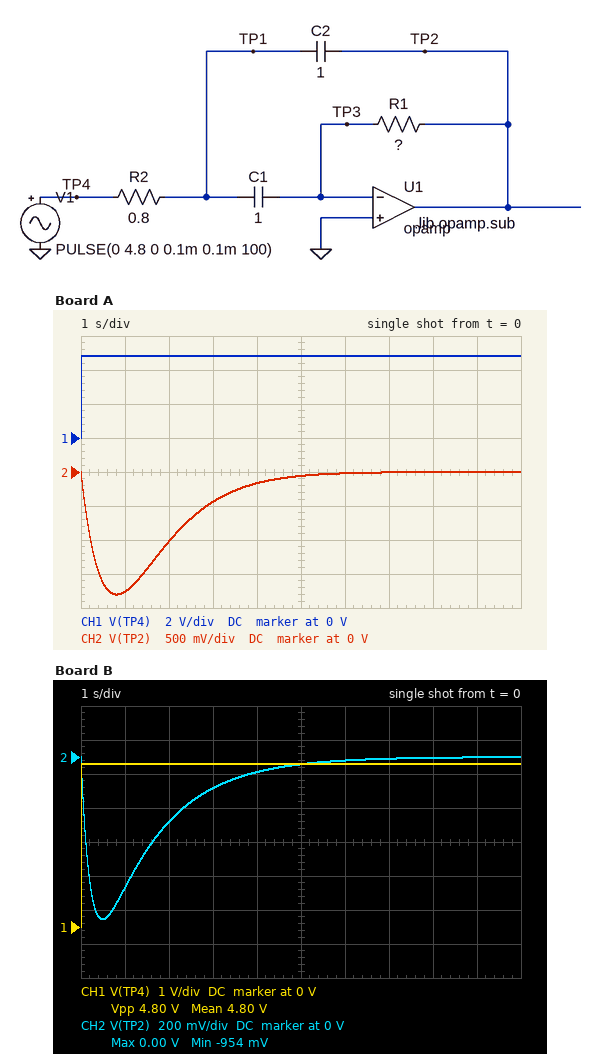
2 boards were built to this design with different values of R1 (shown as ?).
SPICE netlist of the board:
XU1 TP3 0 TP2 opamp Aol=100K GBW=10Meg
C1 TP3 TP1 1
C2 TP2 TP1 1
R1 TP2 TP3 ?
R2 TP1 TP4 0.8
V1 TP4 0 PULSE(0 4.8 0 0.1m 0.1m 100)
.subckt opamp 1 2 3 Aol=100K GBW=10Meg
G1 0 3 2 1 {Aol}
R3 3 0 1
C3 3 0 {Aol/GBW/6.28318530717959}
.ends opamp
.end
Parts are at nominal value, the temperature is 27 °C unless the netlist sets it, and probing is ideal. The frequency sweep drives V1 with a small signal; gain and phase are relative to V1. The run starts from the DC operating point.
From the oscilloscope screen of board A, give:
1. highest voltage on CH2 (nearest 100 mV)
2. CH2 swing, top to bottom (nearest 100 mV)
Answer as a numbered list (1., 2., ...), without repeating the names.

1. 0 V
2. 1.8 V
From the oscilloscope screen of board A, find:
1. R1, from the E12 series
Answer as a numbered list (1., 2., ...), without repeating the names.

1. 0.82 Ω
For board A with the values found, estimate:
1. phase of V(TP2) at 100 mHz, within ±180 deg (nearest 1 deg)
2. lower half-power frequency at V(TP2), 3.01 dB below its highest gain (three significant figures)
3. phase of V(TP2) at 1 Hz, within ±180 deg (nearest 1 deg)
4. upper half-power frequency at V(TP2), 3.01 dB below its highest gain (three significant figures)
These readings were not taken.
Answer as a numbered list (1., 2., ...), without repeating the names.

1. -144 deg
2. 82.1 mHz
3. 112 deg
4. 470 mHz
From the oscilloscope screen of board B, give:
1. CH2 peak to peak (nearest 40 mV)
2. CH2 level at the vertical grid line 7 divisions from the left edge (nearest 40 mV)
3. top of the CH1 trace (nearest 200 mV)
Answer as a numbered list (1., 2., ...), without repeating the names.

1. 960 mV
2. 0 V
3. 4.8 V
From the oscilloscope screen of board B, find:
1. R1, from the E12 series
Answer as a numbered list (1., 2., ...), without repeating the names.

1. 0.39 Ω
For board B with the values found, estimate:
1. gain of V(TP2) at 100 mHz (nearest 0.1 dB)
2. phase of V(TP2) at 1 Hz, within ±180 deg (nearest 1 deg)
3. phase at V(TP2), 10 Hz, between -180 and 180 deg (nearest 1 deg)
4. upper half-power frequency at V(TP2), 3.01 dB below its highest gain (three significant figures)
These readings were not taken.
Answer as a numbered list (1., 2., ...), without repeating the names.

1. -14.7 dB
2. 132 deg
3. 95 deg
4. 906 mHz
